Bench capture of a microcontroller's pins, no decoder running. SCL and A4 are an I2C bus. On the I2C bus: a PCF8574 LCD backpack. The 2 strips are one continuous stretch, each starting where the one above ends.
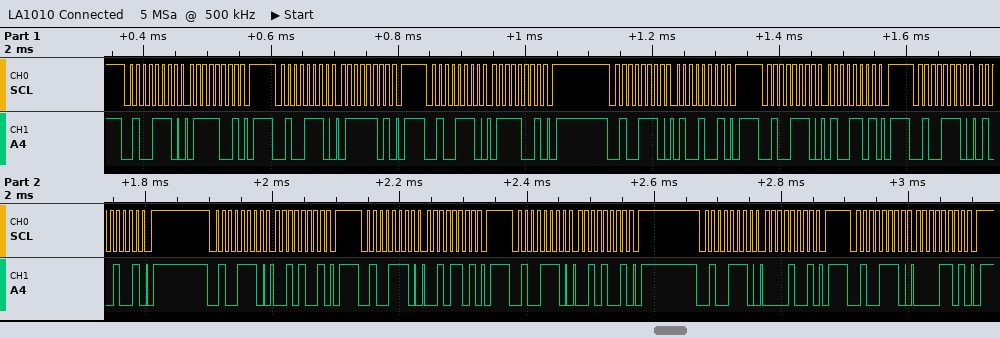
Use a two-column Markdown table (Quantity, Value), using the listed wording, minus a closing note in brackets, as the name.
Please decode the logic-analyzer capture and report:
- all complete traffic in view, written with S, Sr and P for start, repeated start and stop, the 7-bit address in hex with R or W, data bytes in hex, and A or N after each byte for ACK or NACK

| Quantity | Value |
|---|---|
| all complete traffic in view, written with S, Sr and P for start, repeated start and stop, the 7-bit address in hex with R or W, data bytes in hex, and A or N after each byte for ACK or NACK | S 27W A 79 A P S 27W A 7D A P S 27W A 79 A P S 27W A 49 A P S 27W A 4D A P S 27W A 49 A P S 27W A 29 A P S 27W A 2D A P S 27W A 29 A P S 27W A 09 A P S 27W A 0D A P |
